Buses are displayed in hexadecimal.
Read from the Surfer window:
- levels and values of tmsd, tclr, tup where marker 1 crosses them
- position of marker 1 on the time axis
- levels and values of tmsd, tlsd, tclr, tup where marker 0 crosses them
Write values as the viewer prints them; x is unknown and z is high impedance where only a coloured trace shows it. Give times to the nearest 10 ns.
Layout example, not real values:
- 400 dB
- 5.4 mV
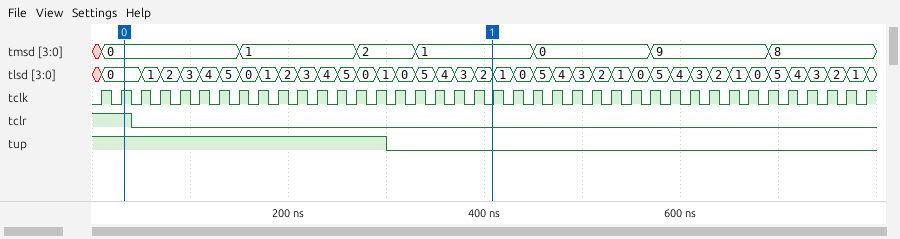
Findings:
- tmsd=1, tclr=0, tup=0
- 410 ns
- tmsd=0, tlsd=0, tclr=1, tup=1
